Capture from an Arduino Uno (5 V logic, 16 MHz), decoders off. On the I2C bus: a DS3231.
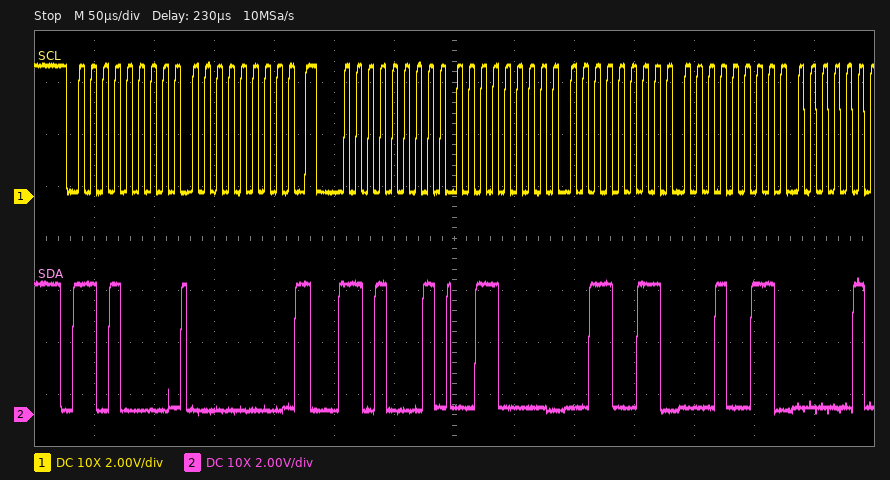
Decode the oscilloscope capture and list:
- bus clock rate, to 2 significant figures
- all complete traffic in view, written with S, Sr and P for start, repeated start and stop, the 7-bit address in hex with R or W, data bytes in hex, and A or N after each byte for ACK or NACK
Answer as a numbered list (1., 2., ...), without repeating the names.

1. 100 kHz
2. S 68W A 00 A Sr 68R A 30 A 33 A 13 A
